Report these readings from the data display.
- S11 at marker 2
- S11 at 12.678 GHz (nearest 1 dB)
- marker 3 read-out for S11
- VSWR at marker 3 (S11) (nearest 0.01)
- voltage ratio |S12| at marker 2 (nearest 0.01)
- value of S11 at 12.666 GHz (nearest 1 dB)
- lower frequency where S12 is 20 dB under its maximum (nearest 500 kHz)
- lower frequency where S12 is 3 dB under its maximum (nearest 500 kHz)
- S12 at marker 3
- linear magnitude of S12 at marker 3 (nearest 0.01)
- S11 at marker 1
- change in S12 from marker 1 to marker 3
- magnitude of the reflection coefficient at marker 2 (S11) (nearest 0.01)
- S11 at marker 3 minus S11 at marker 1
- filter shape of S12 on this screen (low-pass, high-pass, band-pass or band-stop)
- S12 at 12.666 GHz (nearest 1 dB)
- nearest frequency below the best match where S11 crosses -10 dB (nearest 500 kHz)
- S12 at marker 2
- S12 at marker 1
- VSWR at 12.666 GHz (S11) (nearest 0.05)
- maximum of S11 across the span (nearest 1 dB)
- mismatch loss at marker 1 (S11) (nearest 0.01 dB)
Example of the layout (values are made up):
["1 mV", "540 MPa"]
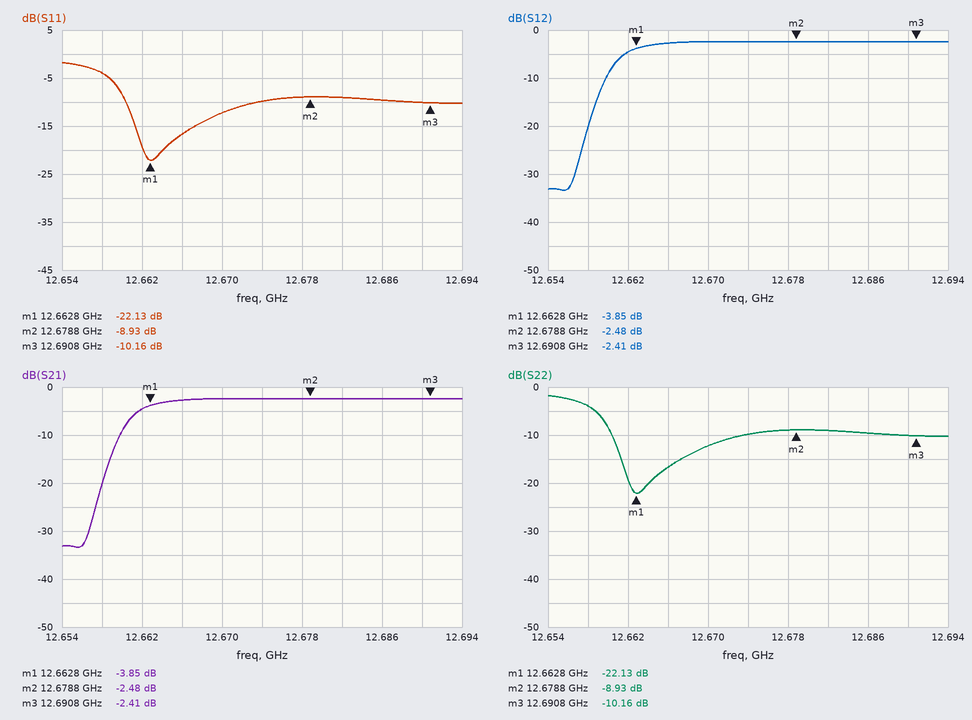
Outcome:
["-8.93 dB", "-9 dB", "-10.16 dB", "1.90", "0.75", "-17 dB", "12.6575 GHz", "12.6615 GHz", "-2.41 dB", "0.76", "-22.13 dB", "1.44 dB", "0.36", "11.97 dB", "high-pass", "-3 dB", "12.6605 GHz", "-2.48 dB", "-3.85 dB", "1.35", "-2 dB", "0.03 dB"]
